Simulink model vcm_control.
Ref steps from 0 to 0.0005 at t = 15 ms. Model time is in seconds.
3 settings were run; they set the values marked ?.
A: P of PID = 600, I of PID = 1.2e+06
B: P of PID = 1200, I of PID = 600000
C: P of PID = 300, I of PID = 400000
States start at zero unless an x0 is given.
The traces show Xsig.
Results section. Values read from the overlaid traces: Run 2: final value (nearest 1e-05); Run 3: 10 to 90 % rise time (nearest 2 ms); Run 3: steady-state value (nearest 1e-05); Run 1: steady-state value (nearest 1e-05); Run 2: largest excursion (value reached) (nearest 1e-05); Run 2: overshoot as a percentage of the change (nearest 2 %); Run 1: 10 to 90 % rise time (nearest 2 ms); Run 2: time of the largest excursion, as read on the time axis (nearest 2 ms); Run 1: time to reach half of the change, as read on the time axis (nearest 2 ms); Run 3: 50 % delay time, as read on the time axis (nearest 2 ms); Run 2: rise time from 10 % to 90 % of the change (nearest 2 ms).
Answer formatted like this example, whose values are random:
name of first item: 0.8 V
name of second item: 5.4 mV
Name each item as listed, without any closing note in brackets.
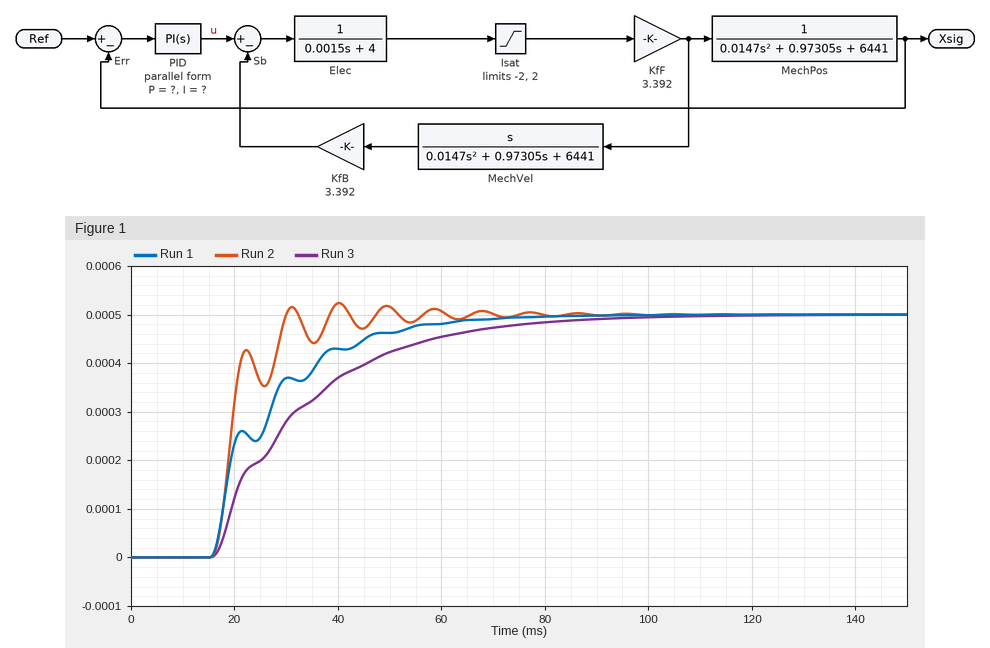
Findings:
Run 2: final value: 0.00050
Run 3: 10 to 90 % rise time: 40 ms
Run 3: steady-state value: 0.00050
Run 1: steady-state value: 0.00050
Run 2: largest excursion (value reached): 0.00052
Run 2: overshoot as a percentage of the change: 4 %
Run 1: 10 to 90 % rise time: 28 ms
Run 2: time of the largest excursion, as read on the time axis: 40 ms
Run 1: time to reach half of the change, as read on the time axis: 20 ms
Run 3: 50 % delay time, as read on the time axis: 28 ms
Run 2: rise time from 10 % to 90 % of the change: 12 ms
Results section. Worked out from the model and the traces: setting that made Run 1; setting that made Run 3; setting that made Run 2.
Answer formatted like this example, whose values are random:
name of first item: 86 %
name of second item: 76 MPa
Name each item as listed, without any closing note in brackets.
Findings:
setting that made Run 1: B
setting that made Run 3: C
setting that made Run 2: A
